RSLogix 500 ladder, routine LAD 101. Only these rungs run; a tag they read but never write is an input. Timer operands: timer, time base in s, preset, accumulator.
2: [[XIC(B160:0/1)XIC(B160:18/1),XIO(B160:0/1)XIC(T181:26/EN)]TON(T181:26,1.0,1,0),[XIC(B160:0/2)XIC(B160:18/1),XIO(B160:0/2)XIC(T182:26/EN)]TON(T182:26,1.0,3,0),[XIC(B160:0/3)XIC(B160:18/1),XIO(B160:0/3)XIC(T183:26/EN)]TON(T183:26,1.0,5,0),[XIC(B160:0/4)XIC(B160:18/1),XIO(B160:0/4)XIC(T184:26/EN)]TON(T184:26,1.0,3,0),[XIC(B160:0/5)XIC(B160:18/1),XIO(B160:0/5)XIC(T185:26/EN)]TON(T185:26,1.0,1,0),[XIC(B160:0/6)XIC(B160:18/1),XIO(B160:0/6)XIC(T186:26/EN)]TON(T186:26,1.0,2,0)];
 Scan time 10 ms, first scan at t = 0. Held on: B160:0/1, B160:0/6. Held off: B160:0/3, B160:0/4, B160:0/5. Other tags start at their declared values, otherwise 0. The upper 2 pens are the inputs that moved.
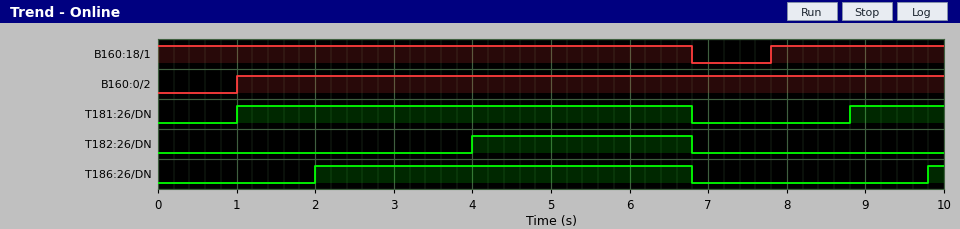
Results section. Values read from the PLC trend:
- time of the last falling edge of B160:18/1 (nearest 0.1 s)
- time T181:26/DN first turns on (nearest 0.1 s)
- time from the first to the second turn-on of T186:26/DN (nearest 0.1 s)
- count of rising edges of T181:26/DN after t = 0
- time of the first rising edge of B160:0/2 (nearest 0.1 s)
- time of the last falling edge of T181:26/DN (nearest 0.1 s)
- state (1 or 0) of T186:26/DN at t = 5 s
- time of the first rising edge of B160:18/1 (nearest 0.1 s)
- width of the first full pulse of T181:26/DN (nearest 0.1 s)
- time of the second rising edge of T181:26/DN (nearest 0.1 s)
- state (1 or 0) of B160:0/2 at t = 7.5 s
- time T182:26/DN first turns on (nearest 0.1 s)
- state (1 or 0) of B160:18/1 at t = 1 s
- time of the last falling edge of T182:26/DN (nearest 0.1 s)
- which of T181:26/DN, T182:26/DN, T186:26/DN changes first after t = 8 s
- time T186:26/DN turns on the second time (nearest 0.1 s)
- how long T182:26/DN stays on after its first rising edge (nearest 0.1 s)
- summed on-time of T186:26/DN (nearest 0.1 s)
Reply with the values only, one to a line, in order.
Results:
6.8 s
1.0 s
7.8 s
2
1.0 s
6.8 s
1
7.8 s
5.8 s
8.8 s
1
4.0 s
1
6.8 s
T181:26/DN
9.8 s
2.8 s
5.0 s
